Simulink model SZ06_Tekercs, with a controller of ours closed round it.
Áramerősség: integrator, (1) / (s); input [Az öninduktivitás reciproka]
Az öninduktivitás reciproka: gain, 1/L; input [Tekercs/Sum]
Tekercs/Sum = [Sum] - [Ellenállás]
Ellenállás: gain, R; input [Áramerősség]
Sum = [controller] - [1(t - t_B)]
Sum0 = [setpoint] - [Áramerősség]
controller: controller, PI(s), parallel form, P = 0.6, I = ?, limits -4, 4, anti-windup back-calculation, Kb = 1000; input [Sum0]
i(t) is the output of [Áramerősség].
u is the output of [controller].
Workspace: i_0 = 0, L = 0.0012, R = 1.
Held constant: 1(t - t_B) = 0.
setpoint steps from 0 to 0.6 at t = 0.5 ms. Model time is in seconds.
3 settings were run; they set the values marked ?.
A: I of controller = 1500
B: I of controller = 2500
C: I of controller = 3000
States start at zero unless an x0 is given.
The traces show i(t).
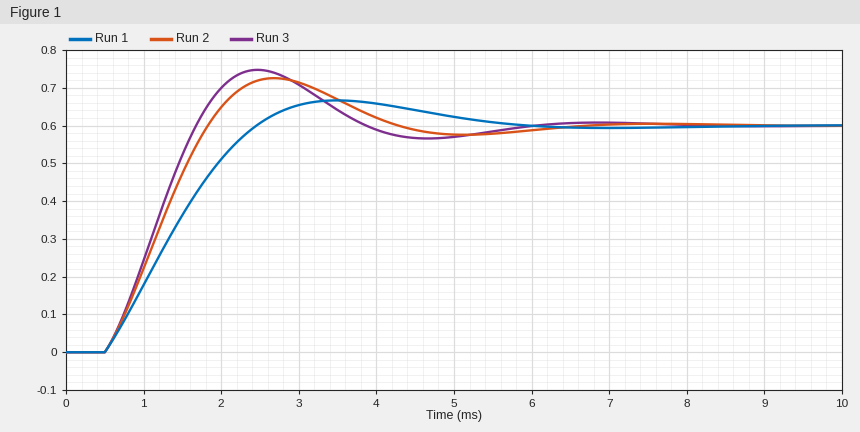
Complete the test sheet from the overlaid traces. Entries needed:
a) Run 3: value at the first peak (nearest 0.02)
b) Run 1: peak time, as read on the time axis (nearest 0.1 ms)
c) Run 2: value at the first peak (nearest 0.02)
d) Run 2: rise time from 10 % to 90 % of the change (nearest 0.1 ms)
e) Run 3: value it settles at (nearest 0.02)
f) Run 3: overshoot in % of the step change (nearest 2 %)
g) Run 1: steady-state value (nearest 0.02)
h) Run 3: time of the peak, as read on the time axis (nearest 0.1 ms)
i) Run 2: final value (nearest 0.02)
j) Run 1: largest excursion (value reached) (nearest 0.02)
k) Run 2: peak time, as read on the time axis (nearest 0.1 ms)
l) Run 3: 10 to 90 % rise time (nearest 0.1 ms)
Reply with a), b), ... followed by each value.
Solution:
a) 0.74
b) 3.5 ms
c) 0.72
d) 1.0 ms
e) 0.60
f) 24 %
g) 0.60
h) 2.5 ms
i) 0.60
j) 0.66
k) 2.7 ms
l) 0.9 ms
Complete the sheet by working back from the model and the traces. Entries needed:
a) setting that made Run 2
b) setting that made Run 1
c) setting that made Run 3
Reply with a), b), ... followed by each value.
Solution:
a) B
b) A
c) C
